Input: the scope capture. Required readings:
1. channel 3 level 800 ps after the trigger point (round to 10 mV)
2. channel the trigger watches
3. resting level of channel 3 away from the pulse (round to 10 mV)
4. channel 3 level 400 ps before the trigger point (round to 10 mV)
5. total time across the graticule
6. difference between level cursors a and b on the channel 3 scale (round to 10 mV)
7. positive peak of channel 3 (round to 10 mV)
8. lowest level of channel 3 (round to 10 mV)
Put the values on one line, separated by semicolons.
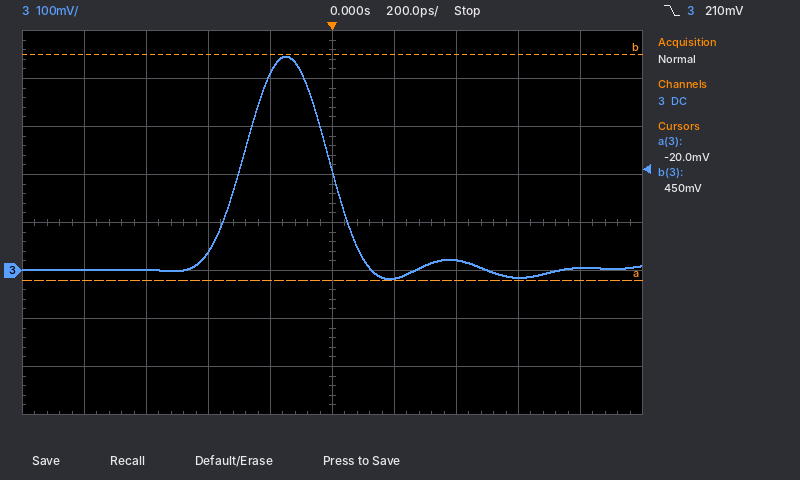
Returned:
10 mV; channel 3; 0 mV; 40 mV; 2 ns; 470 mV; 450 mV; -20 mV
